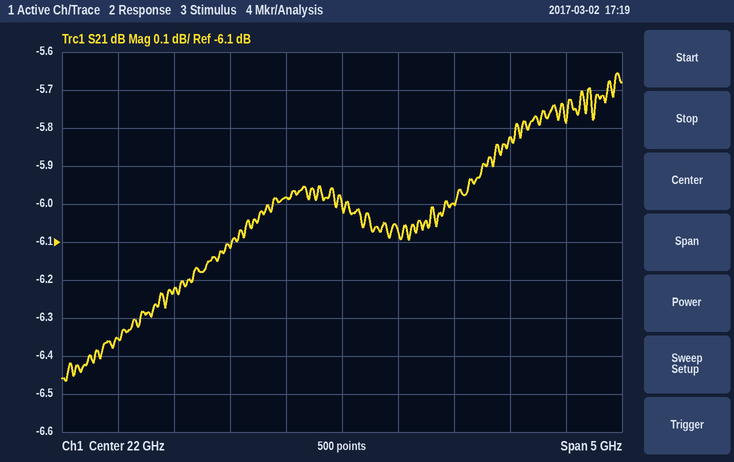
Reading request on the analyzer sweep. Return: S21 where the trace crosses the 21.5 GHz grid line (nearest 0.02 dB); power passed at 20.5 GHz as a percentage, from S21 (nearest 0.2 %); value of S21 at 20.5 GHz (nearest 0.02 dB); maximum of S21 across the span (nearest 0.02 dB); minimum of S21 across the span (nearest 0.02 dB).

-5.98 dB
23.8 %
-6.22 dB
-5.66 dB
-6.46 dB
